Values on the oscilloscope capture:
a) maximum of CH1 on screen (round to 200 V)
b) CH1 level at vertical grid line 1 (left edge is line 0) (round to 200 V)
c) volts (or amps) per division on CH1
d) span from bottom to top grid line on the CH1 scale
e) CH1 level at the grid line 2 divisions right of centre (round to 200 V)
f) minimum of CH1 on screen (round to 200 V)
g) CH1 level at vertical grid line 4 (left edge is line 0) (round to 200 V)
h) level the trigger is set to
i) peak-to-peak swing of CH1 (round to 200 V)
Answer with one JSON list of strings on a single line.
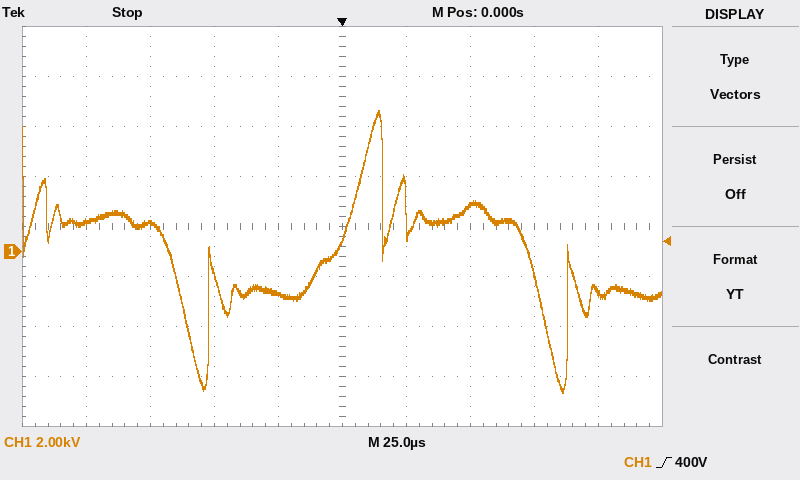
["5.6 kV", "1.2 kV", "2 kV", "16 kV", "1.8 kV", "-5.6 kV", "-1.6 kV", "400 V", "11.2 kV"]
